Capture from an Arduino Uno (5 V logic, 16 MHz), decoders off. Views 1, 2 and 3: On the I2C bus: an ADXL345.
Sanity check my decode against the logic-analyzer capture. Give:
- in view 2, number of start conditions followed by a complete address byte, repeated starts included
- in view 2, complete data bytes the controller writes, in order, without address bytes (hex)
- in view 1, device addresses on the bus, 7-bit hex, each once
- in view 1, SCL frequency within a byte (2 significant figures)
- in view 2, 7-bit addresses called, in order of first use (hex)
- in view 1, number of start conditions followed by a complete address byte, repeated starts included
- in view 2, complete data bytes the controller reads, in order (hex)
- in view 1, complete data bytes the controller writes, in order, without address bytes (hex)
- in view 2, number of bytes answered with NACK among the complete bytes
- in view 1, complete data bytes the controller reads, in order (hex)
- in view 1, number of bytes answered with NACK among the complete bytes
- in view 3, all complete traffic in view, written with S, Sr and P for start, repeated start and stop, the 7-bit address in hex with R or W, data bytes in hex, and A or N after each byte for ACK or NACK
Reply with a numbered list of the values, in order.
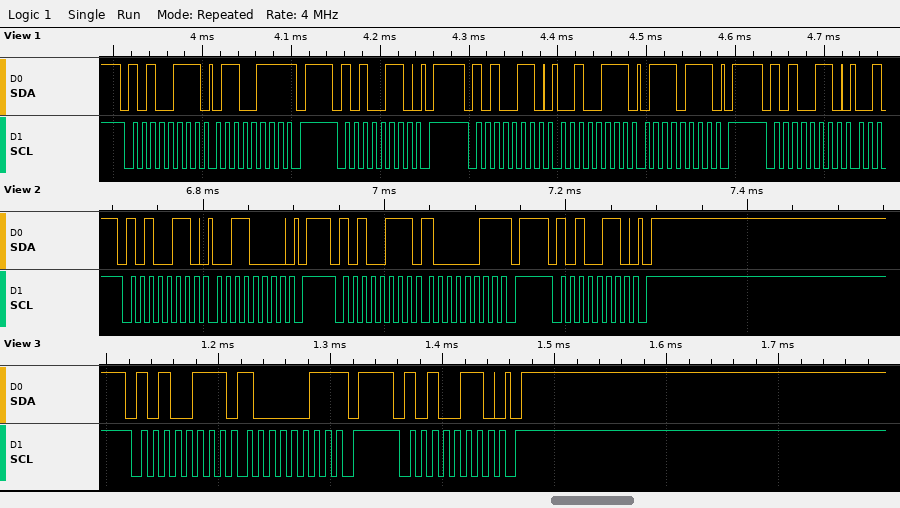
1. 3
2. 30
3. 0x53
4. 100 kHz
5. 0x53
6. 4
7. 83
8. 27 77
9. 1
10. 67
11. 1
12. S 53R A 83 N P S 53W A P
